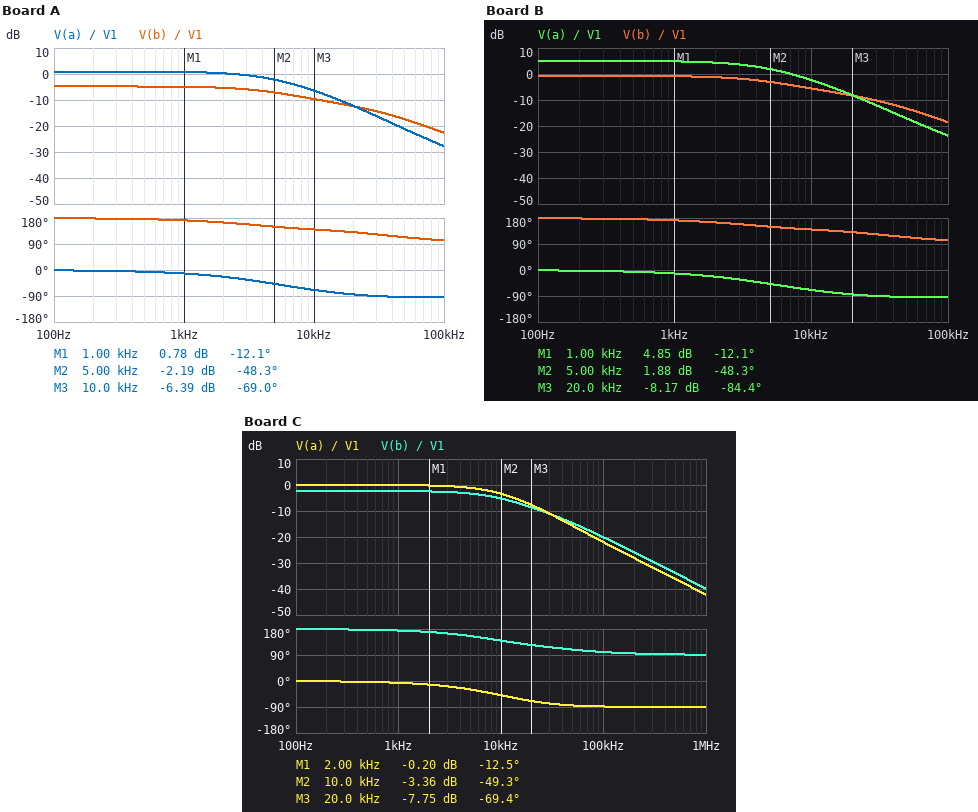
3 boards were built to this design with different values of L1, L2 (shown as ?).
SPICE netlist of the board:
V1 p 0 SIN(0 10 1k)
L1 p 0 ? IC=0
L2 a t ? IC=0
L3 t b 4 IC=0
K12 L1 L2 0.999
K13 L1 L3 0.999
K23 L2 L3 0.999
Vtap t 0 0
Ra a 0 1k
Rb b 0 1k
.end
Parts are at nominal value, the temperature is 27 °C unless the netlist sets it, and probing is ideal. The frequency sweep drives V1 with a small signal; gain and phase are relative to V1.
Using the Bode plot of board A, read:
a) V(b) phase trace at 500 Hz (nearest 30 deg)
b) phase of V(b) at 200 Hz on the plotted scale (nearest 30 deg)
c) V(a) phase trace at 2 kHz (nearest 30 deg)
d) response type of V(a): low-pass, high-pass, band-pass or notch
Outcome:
180 deg
180 deg
-30 deg
low-pass
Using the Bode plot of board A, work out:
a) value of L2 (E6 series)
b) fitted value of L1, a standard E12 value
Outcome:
15 H
12 H
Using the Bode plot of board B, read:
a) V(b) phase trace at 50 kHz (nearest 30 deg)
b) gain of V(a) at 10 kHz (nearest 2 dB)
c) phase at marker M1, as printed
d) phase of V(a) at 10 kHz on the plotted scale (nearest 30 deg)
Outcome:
120 deg
-2 dB
-12.1 deg
-60 deg
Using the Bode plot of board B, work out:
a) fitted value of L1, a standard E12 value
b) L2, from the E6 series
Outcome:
4.7 H
15 H
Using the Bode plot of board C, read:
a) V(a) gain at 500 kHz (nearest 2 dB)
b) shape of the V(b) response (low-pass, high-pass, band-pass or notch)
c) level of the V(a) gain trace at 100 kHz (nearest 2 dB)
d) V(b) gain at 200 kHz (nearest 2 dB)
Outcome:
-36 dB
low-pass
-22 dB
-26 dB
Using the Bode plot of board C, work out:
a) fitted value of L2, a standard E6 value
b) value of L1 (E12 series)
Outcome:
6.8 H
6.8 H
